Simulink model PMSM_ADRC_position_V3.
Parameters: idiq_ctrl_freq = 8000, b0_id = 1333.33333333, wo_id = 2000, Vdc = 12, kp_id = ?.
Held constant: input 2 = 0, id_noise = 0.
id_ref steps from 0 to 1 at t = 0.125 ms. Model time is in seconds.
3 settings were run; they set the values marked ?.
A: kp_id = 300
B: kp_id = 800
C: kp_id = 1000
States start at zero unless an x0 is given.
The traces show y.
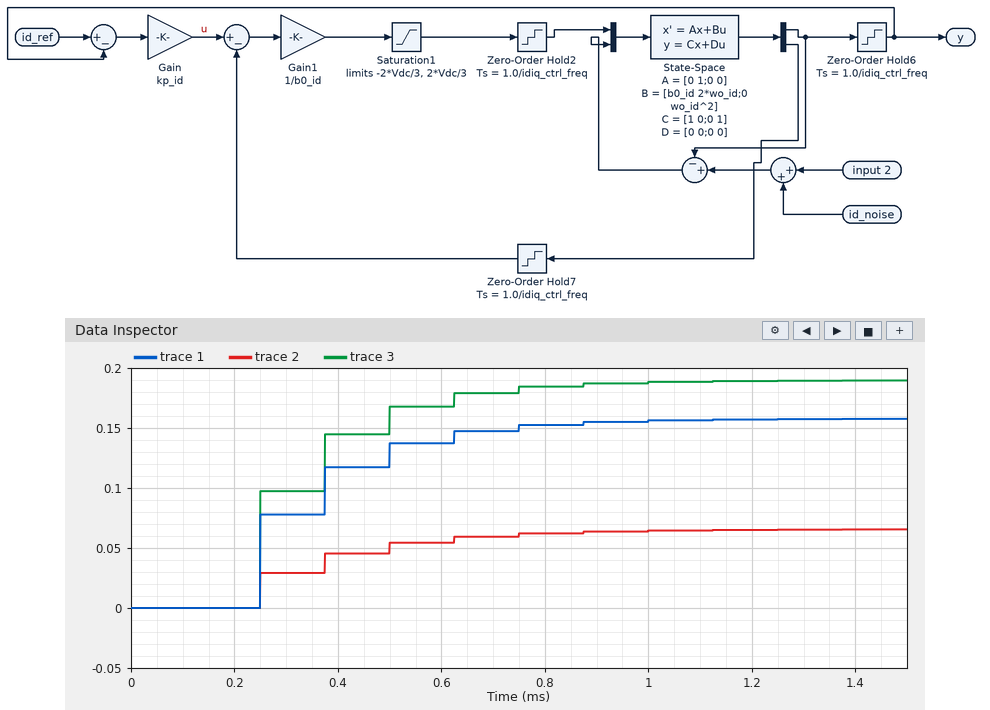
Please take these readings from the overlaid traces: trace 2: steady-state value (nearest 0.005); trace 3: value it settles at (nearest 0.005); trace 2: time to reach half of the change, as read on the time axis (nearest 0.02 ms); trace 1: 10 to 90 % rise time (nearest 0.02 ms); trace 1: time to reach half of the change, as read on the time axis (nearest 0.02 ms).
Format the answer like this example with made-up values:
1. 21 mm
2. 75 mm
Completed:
1. 0.065
2. 0.190
3. 0.38 ms
4. 0.38 ms
5. 0.38 ms
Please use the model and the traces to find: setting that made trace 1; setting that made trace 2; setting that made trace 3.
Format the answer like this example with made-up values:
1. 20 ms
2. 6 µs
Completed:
1. B
2. A
3. C
